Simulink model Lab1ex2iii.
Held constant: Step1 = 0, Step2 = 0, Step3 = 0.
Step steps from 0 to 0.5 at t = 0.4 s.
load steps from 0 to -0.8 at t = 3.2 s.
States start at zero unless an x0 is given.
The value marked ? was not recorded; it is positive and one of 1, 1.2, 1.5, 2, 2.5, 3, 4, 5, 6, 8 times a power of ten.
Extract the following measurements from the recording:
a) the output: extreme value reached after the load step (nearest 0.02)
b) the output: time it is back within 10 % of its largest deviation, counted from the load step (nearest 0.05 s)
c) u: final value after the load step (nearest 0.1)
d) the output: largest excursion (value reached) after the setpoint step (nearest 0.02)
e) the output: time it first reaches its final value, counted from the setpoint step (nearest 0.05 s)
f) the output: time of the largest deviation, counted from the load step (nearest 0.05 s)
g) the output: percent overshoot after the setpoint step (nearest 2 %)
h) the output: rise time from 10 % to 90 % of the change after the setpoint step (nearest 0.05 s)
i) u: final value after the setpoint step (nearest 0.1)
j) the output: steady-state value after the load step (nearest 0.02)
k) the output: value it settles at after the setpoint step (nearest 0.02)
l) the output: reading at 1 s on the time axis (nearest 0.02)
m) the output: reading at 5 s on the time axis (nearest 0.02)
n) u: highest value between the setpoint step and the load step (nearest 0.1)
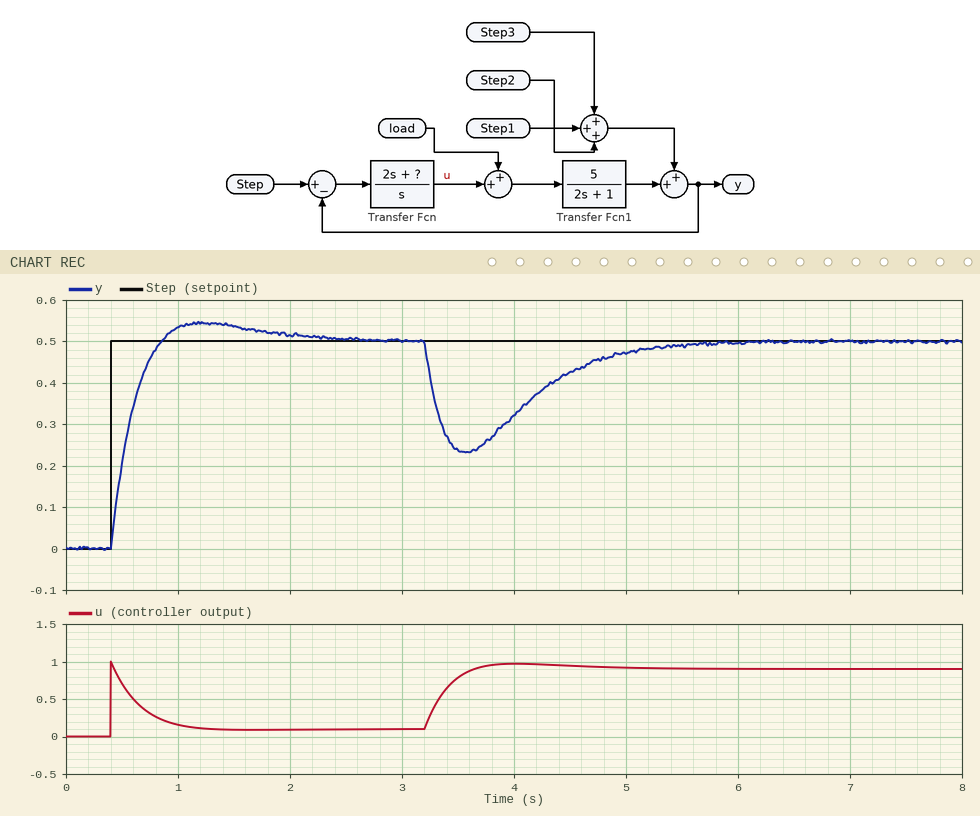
0.24
1.80 s
0.9
0.54
0.45 s
0.35 s
8 %
0.30 s
0.1
0.50
0.50
0.54
0.48
1.0
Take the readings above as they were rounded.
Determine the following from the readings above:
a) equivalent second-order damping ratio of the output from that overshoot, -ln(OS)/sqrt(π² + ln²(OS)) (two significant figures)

0.63
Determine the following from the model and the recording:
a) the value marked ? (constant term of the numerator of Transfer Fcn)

3
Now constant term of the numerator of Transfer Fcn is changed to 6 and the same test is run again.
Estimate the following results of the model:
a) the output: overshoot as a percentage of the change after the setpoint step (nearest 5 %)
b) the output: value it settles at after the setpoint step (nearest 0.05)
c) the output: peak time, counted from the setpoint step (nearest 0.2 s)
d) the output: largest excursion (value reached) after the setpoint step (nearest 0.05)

15 %
0.50
0.6 s
0.60
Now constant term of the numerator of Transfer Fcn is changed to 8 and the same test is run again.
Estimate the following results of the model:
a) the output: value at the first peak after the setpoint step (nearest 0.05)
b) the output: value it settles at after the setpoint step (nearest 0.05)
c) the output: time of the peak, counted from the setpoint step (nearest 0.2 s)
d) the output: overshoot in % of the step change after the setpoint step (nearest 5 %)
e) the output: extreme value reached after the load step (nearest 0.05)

0.60
0.50
0.6 s
20 %
0.30
